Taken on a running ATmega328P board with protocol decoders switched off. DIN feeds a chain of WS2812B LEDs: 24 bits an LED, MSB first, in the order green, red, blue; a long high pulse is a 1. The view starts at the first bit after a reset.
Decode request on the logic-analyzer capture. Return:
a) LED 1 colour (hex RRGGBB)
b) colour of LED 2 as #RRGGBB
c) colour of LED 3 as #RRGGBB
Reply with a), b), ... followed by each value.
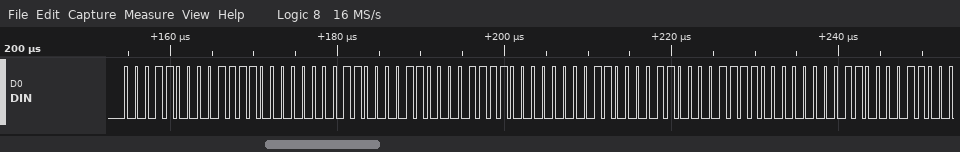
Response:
a) #781806
b) #781806
c) #781806
